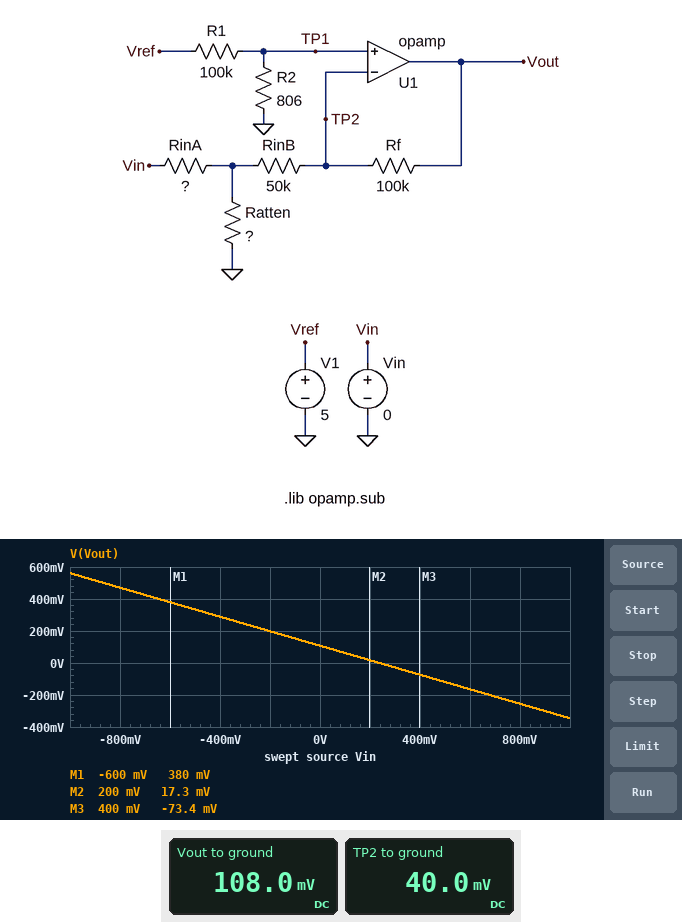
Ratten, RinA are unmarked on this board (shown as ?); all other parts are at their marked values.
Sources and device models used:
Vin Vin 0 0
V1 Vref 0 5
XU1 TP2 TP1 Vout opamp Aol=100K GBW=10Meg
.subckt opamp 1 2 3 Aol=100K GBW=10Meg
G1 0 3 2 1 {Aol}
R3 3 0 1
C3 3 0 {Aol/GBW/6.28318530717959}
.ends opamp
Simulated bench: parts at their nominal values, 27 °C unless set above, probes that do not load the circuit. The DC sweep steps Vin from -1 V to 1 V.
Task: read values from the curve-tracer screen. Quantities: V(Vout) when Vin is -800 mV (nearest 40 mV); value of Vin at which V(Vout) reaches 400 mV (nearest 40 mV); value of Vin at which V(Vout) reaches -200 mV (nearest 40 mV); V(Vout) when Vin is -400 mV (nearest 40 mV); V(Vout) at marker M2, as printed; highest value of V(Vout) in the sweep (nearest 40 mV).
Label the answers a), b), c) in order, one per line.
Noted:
a) 480 mV
b) -640 mV
c) 680 mV
d) 280 mV
e) 17.3 mV
f) 560 mV
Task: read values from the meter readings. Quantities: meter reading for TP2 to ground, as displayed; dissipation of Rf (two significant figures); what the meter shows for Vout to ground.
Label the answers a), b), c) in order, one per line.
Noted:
a) 40.0 mV
b) 46 nW
c) 108.0 mV
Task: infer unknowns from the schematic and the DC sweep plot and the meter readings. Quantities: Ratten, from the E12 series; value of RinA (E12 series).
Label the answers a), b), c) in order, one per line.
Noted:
a) 12 kΩ
b) 33 kΩ
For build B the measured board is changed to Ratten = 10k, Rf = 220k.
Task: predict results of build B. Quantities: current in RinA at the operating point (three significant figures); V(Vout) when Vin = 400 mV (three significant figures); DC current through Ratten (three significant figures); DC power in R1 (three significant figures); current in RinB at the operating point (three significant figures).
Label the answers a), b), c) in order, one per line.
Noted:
a) 161 nA
b) -162 mV
c) 532 nA
d) 246 µW
e) 693 nA
